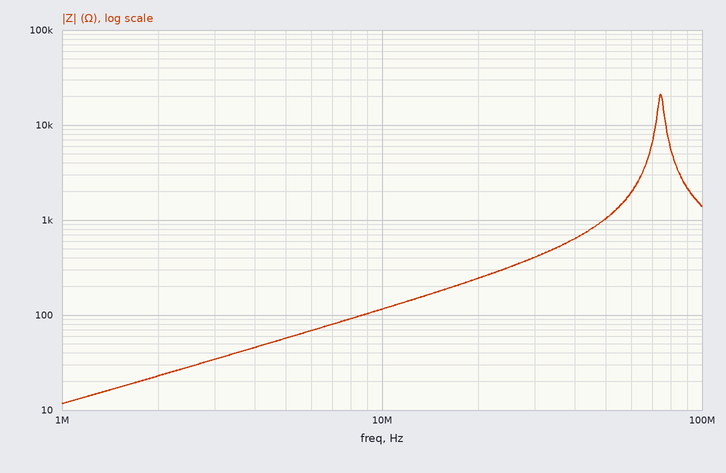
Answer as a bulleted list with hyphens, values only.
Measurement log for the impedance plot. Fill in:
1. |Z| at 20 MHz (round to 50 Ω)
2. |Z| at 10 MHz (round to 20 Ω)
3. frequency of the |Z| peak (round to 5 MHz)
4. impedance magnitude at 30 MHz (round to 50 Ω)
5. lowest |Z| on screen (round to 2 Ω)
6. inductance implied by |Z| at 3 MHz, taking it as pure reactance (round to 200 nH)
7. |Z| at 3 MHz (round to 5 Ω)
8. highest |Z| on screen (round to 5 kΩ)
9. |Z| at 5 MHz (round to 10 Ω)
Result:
- 250 Ω
- 120 Ω
- 75 MHz
- 400 Ω
- 12 Ω
- 1.8 µH
- 35 Ω
- 20 kΩ
- 60 Ω
